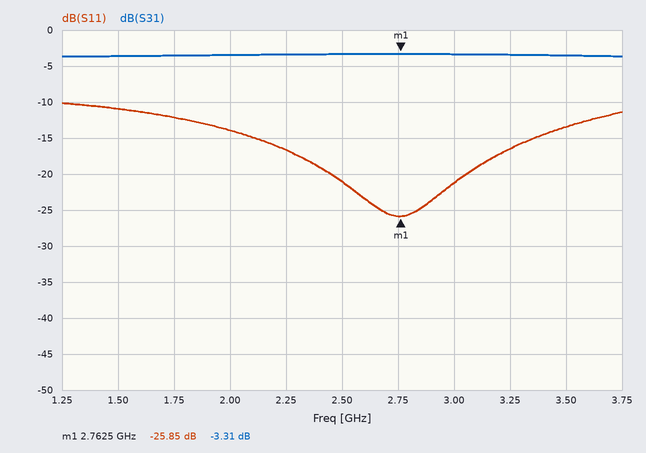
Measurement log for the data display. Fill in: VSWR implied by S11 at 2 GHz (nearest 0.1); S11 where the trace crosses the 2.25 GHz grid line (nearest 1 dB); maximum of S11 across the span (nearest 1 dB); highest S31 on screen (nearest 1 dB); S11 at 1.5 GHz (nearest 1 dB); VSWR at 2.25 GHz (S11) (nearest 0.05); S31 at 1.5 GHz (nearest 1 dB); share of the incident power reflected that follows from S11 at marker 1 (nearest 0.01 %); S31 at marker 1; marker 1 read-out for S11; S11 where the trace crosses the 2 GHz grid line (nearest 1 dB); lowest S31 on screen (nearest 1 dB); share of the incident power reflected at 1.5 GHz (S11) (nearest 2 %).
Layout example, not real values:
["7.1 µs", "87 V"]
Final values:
["1.5", "-17 dB", "-10 dB", "-3 dB", "-11 dB", "1.35", "-4 dB", "0.26 %", "-3.31 dB", "-25.85 dB", "-14 dB", "-4 dB", "8 %"]
